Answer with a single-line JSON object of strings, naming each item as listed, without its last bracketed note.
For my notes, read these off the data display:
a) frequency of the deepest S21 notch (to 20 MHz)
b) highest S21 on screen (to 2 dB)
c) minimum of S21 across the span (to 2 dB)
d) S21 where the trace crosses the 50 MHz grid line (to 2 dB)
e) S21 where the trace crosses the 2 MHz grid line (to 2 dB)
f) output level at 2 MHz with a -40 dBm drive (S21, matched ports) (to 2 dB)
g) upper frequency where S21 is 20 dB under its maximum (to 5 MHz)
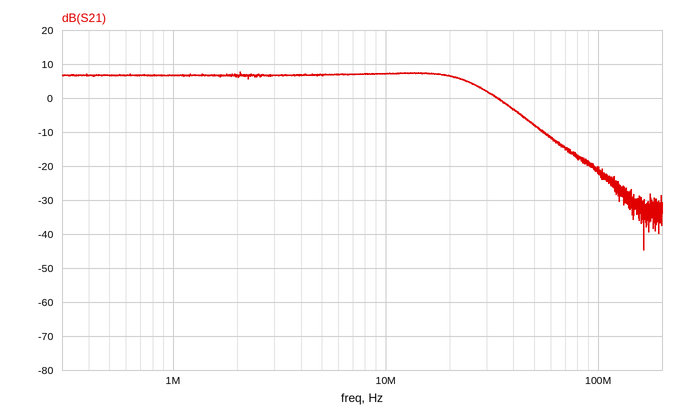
{"frequency of the deepest S21 notch": "160 MHz", "highest S21 on screen": "8 dB", "minimum of S21 across the span": "-44 dB", "S21 where the trace crosses the 50 MHz grid line": "-8 dB", "S21 where the trace crosses the 2 MHz grid line": "6 dB", "output level at 2 MHz with a -40 dBm drive (S21, matched ports)": "-34 dBm", "upper frequency where S21 is 20 dB under its maximum": "60 MHz"}
